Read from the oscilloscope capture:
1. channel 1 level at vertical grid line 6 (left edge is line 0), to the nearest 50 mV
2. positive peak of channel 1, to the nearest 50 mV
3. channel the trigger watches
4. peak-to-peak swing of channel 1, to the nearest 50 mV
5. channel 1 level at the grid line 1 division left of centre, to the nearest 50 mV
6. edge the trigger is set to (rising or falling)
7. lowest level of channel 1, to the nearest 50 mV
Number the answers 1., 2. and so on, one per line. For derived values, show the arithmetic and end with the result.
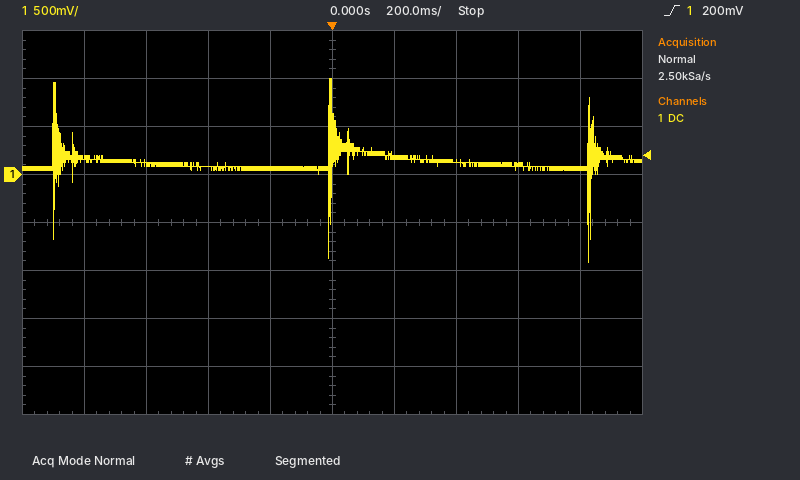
1. 200 mV
2. 1.00 V
3. channel 1
4. 1.00 V − (-900 mV) = 1.90 V
5. 50 mV
6. rising
7. -900 mV
